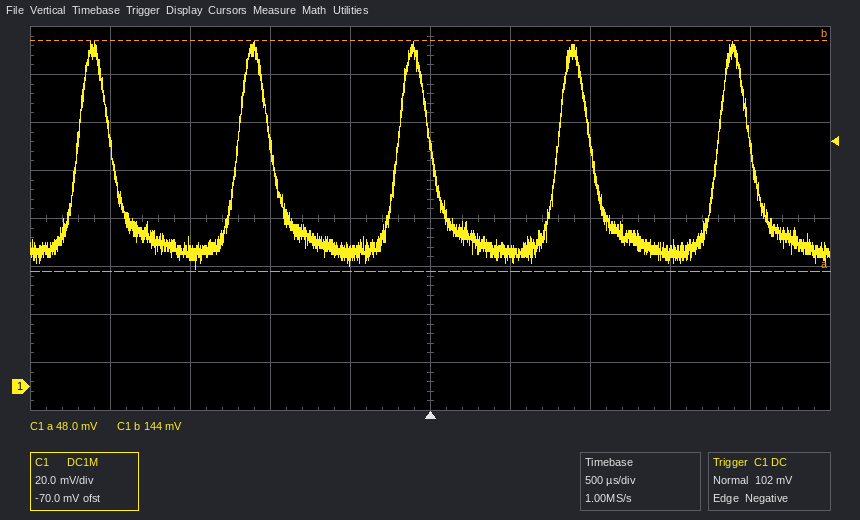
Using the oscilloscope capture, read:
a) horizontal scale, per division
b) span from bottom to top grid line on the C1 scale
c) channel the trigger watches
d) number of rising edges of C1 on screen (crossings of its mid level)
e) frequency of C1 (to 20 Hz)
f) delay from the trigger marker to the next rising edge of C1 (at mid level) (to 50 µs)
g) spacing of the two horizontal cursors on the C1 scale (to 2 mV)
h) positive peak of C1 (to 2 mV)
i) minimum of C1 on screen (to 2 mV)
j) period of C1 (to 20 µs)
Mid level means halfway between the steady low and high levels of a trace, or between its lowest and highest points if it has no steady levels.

500 µs
160 mV
C1
5
1.00 kHz
800 µs
96 mV
144 mV
48 mV
1.00 ms
